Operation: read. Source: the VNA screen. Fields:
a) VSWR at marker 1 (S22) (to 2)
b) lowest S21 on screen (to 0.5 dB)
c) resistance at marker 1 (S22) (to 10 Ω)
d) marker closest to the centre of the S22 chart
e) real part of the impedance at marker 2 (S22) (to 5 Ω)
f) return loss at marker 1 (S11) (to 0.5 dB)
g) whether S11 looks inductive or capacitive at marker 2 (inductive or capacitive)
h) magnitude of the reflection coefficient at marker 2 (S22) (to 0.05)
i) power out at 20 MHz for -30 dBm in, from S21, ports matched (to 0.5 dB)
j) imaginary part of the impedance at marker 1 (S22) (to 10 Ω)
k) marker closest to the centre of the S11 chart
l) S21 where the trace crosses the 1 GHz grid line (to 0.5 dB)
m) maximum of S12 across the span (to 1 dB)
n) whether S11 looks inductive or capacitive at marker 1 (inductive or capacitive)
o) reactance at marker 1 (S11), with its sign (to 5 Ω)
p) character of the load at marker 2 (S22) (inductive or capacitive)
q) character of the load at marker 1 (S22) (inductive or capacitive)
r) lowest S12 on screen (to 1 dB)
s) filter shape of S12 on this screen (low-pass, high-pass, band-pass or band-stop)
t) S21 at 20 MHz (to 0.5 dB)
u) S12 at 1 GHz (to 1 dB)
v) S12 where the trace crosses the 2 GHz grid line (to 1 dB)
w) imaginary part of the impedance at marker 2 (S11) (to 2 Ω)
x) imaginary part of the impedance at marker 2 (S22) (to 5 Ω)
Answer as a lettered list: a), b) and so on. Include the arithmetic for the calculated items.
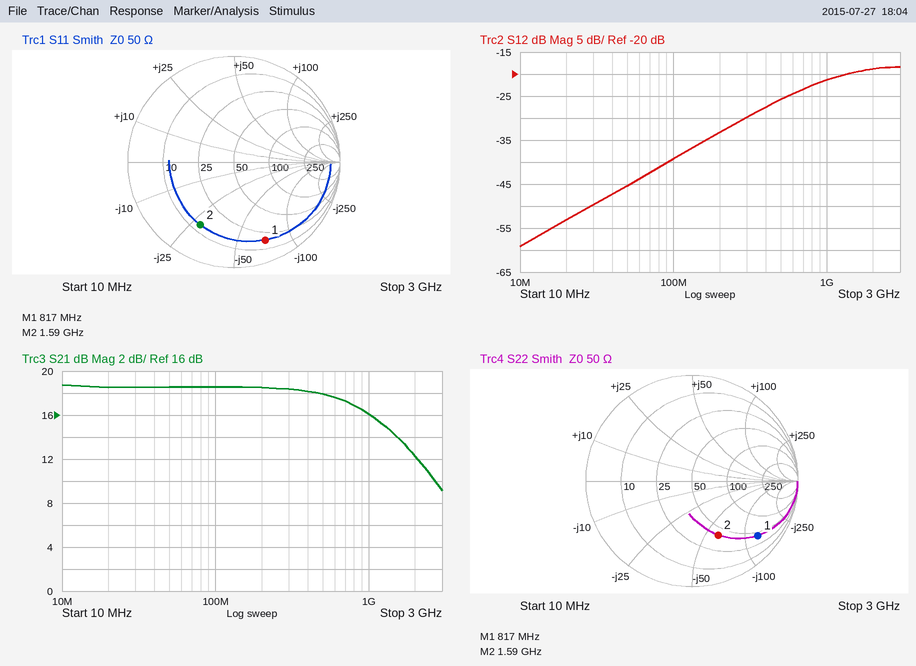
a) 10
b) 9.0 dB
c) 40 Ω
d) marker 2
e) 40 Ω
f) 2.0 dB
g) capacitive
h) 0.55
i) -30 dBm + (18.5 dB) = -11.5 dBm
j) -130 Ω
k) marker 2
l) 16.0 dB
m) -18 dB
n) capacitive
o) -70 Ω
p) capacitive
q) capacitive
r) -59 dB
s) high-pass
t) 18.5 dB
u) -21 dB
v) -19 dB
w) -28 Ω
x) -60 Ω
